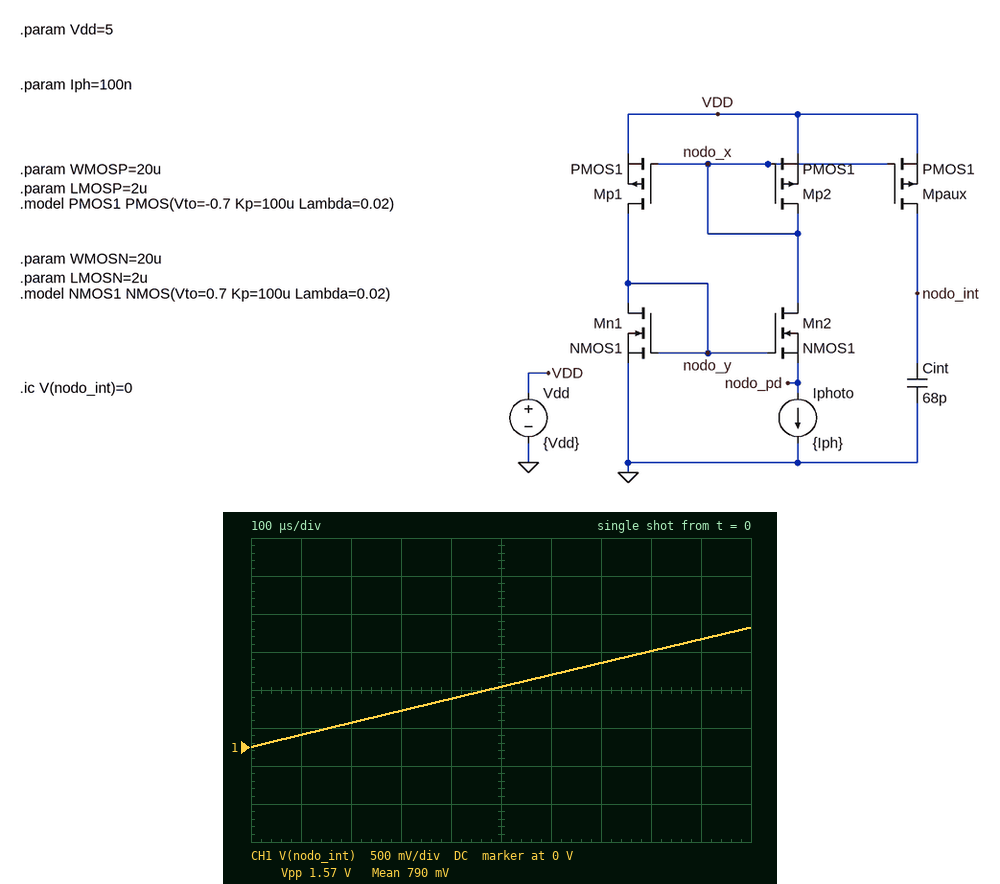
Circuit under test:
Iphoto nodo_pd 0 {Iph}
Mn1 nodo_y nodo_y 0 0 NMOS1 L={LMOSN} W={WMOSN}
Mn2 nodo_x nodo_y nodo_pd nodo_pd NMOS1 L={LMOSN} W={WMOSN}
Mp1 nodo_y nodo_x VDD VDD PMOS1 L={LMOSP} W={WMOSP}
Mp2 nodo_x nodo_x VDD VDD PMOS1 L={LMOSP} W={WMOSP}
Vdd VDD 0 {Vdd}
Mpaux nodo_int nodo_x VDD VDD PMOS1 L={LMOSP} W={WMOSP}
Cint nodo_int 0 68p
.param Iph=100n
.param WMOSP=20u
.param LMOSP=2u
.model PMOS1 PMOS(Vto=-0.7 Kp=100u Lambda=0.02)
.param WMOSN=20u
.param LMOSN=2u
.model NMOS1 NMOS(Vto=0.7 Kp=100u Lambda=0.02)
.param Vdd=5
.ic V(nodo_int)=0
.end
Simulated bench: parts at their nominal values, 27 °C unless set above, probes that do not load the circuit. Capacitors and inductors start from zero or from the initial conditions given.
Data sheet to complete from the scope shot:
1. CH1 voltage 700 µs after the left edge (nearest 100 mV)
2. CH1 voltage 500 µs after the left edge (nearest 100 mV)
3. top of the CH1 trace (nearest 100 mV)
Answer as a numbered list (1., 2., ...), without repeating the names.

1. 1.1 V
2. 800 mV
3. 1.6 V
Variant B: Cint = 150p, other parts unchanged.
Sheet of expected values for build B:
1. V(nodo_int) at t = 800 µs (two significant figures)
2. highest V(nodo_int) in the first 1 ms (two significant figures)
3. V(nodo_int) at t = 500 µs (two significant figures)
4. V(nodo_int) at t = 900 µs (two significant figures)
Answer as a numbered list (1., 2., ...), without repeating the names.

1. 580 mV
2. 720 mV
3. 360 mV
4. 650 mV
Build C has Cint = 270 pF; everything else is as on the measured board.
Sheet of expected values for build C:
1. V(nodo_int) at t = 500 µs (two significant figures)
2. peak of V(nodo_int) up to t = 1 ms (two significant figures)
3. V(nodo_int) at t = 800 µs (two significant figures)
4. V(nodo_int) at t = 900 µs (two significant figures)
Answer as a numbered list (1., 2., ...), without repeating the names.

1. 200 mV
2. 400 mV
3. 320 mV
4. 360 mV
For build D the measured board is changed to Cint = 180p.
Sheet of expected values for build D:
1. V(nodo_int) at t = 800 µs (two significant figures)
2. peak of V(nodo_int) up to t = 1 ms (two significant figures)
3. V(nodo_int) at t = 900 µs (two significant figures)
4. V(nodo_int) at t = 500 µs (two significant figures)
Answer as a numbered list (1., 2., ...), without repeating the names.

1. 480 mV
2. 600 mV
3. 540 mV
4. 300 mV
